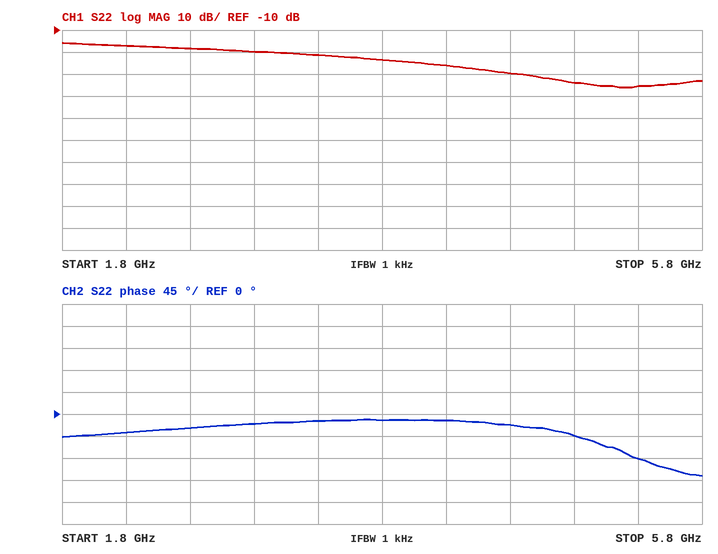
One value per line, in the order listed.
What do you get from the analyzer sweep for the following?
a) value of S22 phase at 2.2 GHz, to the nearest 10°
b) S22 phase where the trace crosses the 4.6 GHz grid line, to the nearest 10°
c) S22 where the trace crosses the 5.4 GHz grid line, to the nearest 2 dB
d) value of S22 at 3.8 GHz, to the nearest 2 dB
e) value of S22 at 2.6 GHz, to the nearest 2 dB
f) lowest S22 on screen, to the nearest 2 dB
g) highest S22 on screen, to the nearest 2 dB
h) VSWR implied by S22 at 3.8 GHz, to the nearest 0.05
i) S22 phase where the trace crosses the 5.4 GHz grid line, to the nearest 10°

-40°
-20°
-36 dB
-24 dB
-18 dB
-36 dB
-16 dB
1.15
-90°
